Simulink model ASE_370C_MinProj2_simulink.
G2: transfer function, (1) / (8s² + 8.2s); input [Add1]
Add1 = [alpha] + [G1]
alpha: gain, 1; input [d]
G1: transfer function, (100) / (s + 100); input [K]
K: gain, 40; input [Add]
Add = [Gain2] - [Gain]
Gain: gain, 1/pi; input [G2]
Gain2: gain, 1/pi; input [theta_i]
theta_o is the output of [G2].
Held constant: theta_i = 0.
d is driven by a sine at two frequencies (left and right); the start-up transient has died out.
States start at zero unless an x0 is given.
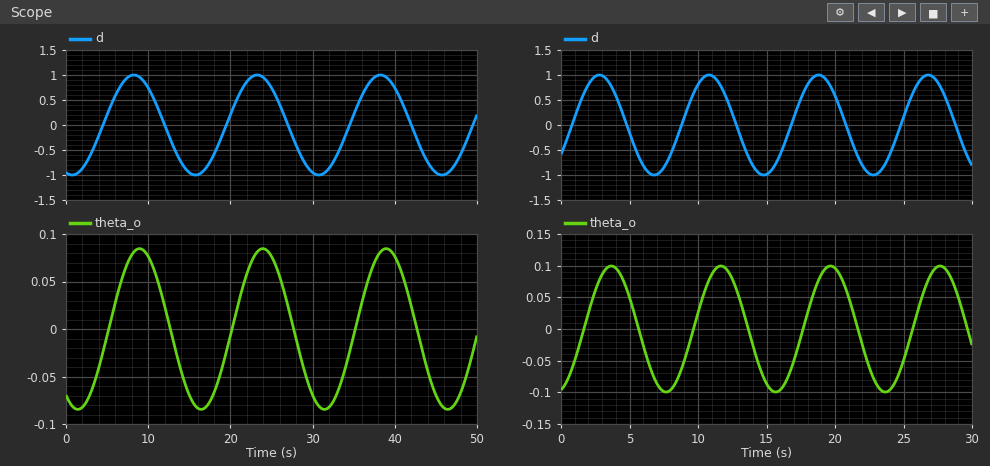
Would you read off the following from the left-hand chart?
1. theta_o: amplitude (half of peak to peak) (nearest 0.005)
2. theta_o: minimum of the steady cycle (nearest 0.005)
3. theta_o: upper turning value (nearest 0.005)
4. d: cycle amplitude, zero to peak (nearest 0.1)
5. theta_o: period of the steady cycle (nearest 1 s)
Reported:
0.085
-0.085
0.085
1.0
15 s
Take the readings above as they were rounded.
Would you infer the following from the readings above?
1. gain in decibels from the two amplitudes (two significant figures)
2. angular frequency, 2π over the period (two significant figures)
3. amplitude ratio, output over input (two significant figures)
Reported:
-21 dB
0.42 rad/s
0.085
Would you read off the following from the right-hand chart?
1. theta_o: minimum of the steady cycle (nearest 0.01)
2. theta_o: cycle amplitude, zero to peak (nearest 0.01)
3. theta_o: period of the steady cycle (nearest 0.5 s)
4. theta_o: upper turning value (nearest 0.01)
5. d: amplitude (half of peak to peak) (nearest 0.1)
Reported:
-0.10
0.10
8.0 s
0.10
1.0
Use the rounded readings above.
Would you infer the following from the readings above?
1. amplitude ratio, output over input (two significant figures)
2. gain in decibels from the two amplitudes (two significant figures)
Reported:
0.10
-20 dB
